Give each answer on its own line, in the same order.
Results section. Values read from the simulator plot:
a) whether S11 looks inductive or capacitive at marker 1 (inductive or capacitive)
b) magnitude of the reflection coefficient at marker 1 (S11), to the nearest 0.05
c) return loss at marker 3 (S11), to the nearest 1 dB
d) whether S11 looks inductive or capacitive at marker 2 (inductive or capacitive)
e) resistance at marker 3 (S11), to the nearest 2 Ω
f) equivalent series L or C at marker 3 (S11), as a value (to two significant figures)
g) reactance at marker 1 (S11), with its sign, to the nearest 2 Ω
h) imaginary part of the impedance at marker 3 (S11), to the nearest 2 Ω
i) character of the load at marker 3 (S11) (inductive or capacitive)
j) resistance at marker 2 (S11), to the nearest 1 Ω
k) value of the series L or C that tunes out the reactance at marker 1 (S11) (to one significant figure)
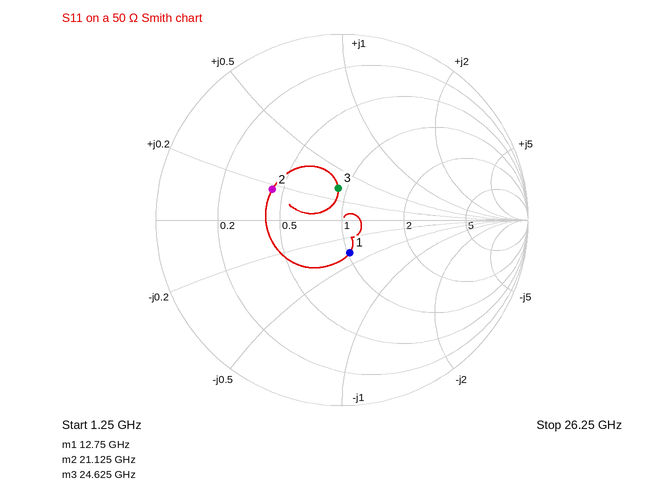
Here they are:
capacitive
0.20
15 dB
inductive
46 Ω
100 pH
-18 Ω
+16 Ω
inductive
22 Ω
200 pH
